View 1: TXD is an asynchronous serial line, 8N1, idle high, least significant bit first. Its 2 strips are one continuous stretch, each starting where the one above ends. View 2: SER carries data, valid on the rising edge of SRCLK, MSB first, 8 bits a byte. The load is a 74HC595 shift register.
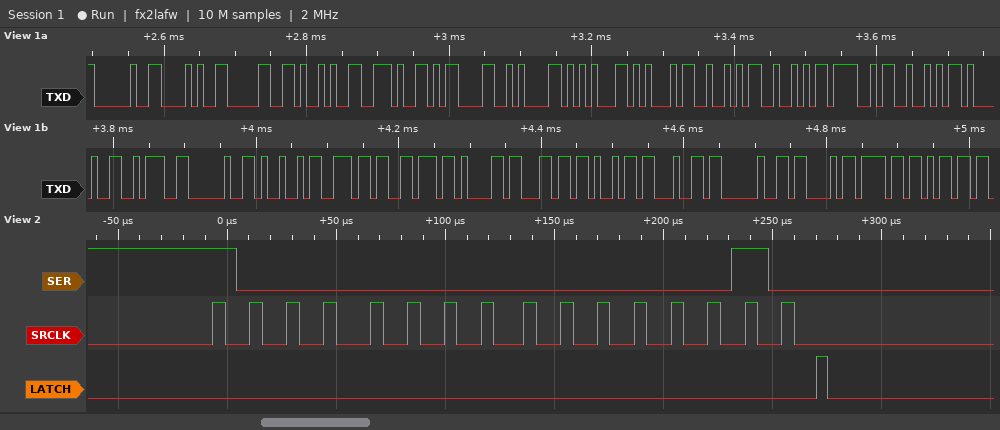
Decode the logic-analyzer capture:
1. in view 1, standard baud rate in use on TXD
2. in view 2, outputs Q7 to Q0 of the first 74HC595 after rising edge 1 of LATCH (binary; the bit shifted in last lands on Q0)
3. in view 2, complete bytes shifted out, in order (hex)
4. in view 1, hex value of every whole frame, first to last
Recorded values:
115200 baud
00000010
80 02
20 28 30 29 2E 0D 0A 15 45 52 52 4F 52 21 3A 20 49 6E 76 61 6C 69 64 20 43 6F 6D
